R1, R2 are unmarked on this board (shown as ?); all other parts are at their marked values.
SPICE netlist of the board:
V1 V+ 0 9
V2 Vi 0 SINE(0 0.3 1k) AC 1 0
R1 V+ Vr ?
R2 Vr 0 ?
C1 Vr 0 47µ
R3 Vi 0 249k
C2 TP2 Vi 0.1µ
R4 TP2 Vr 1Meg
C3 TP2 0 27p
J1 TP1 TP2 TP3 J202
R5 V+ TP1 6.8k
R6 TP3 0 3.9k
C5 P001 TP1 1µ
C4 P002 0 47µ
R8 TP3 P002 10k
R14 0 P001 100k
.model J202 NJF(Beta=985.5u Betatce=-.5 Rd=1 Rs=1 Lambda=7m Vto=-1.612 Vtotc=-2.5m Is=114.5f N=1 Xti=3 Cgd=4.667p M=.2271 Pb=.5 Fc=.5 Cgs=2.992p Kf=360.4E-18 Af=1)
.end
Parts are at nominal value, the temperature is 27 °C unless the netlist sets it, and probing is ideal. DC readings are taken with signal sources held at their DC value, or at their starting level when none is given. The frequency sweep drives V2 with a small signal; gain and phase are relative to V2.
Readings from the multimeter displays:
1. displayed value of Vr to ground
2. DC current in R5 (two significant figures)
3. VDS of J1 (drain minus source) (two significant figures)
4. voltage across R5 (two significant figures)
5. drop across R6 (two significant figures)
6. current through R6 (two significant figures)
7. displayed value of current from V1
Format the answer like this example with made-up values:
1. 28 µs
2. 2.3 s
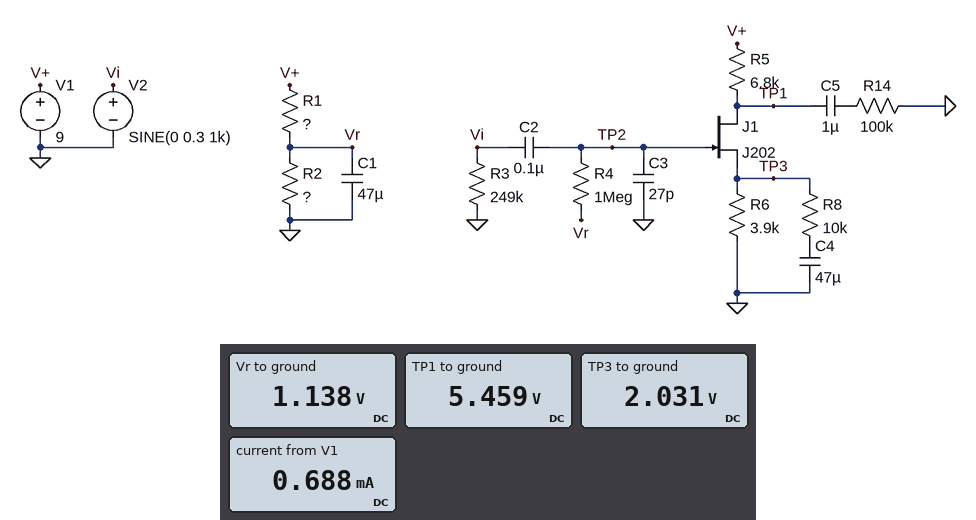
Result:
1. 1.138 V
2. 520 µA
3. 3.4 V
4. 3.5 V
5. 2.0 V
6. 520 µA
7. 0.688 mA
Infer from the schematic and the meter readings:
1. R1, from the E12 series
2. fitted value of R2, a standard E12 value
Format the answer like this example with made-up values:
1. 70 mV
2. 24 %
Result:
1. 47 kΩ
2. 6.8 kΩ
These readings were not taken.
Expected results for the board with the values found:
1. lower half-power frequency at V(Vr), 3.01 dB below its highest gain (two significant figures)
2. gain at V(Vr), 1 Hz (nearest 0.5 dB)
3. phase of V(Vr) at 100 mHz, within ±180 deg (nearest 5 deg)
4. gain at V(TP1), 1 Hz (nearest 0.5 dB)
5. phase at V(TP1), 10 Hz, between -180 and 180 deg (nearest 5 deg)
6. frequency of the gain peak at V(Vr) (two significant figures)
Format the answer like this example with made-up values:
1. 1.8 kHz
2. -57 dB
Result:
1. 360 mHz
2. -56.0 dB
3. 75 deg
4. 0 dB
5. -170 deg
6. 950 mHz
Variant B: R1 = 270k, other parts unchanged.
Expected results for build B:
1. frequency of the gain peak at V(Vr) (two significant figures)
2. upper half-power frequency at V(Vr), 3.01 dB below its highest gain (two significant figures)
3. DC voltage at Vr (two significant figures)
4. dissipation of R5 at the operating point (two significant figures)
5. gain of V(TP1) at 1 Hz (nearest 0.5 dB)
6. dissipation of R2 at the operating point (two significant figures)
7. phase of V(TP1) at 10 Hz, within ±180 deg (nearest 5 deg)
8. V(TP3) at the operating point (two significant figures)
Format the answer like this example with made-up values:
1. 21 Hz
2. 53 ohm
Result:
1. 900 mHz
2. 2.4 Hz
3. 220 mV
4. 720 µW
5. -0.5 dB
6. 7.2 µW
7. -170 deg
8. 1.3 V
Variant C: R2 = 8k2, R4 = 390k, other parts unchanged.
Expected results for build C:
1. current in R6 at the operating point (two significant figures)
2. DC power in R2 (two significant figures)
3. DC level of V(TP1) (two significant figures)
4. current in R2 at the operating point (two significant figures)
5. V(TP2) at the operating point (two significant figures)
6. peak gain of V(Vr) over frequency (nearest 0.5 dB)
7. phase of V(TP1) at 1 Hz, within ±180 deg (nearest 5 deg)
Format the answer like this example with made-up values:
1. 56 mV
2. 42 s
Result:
1. 560 µA
2. 220 µW
3. 5.2 V
4. 160 µA
5. 1.3 V
6. -54.5 dB
7. -100 deg
